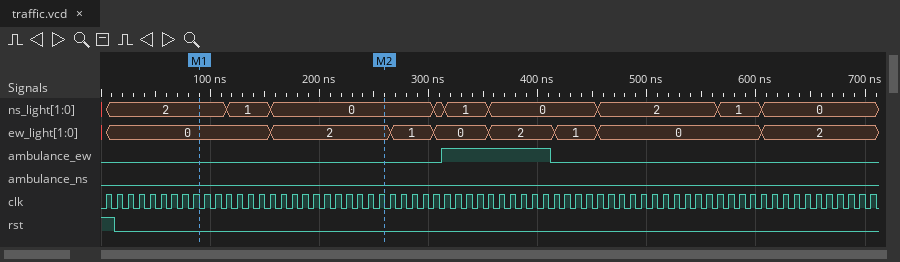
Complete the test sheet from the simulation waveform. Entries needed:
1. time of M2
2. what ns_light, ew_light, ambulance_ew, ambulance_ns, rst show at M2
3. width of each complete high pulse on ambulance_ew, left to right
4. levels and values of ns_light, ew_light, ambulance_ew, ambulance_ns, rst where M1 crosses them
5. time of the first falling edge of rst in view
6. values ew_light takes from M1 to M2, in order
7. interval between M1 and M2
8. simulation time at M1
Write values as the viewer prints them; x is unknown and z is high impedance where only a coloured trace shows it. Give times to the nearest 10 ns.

260 ns
ns_light=0, ew_light=2, ambulance_ew=0, ambulance_ns=0, rst=0
100 ns
ns_light=2, ew_light=0, ambulance_ew=0, ambulance_ns=0, rst=0
10 ns
0, 2
170 ns
90 ns
